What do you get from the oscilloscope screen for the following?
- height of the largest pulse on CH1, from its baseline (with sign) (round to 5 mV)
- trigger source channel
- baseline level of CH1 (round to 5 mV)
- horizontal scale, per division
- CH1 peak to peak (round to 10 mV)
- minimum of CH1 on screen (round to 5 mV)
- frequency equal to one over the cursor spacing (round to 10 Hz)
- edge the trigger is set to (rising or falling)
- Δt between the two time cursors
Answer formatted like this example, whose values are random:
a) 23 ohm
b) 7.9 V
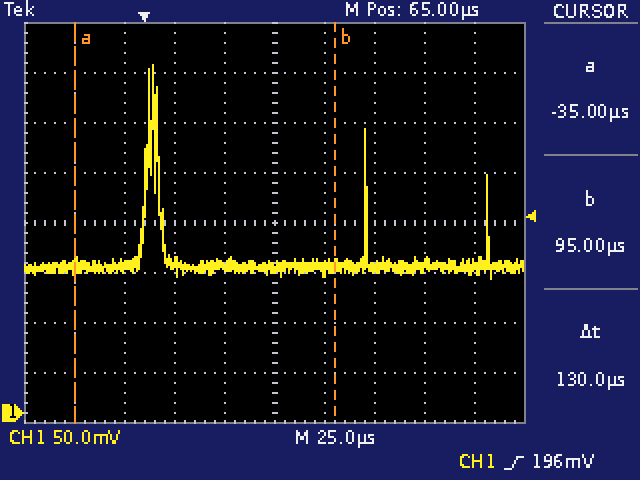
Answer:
a) +200 mV
b) CH1
c) 145 mV
d) 25 µs
e) 210 mV
f) 135 mV
g) 7.69 kHz
h) rising
i) 130 µs
